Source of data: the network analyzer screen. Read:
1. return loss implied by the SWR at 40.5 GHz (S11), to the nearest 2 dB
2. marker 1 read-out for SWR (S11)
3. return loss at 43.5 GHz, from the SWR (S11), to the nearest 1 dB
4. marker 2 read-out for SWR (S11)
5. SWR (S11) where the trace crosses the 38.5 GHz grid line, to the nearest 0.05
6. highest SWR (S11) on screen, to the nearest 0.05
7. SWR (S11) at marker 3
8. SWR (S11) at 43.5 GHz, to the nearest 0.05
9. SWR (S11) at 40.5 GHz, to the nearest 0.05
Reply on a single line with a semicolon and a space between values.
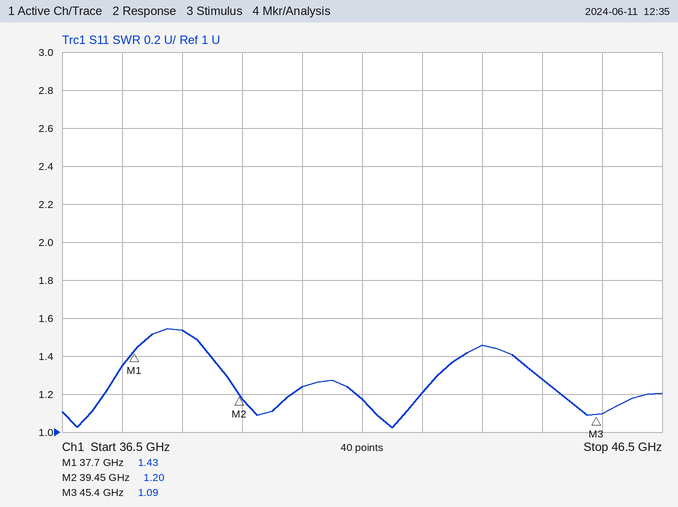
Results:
20 dB; 1.43; 15 dB; 1.20; 1.55; 1.55; 1.09; 1.45; 1.25
